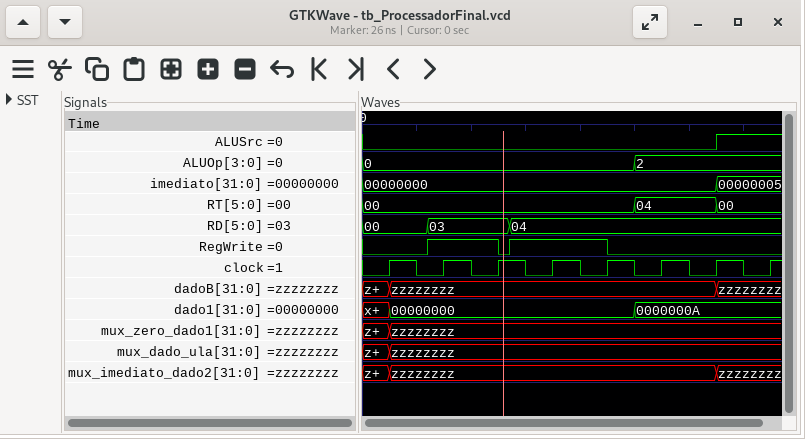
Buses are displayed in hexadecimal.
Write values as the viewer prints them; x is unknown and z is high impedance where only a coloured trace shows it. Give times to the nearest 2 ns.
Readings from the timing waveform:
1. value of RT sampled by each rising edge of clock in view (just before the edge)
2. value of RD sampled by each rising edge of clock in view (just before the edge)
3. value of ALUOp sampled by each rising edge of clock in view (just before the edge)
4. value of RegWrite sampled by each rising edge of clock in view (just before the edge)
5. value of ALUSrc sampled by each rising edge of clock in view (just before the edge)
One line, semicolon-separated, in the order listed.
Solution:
00, 00, 00, 00, 00, 04, 04, 00; 00, 03, 03, 04, 04, 04, 04, 04; 0, 0, 0, 0, 0, 2, 2, 2; 0 1 1 1 1 0 0 0; 0 0 0 0 0 0 0 1
